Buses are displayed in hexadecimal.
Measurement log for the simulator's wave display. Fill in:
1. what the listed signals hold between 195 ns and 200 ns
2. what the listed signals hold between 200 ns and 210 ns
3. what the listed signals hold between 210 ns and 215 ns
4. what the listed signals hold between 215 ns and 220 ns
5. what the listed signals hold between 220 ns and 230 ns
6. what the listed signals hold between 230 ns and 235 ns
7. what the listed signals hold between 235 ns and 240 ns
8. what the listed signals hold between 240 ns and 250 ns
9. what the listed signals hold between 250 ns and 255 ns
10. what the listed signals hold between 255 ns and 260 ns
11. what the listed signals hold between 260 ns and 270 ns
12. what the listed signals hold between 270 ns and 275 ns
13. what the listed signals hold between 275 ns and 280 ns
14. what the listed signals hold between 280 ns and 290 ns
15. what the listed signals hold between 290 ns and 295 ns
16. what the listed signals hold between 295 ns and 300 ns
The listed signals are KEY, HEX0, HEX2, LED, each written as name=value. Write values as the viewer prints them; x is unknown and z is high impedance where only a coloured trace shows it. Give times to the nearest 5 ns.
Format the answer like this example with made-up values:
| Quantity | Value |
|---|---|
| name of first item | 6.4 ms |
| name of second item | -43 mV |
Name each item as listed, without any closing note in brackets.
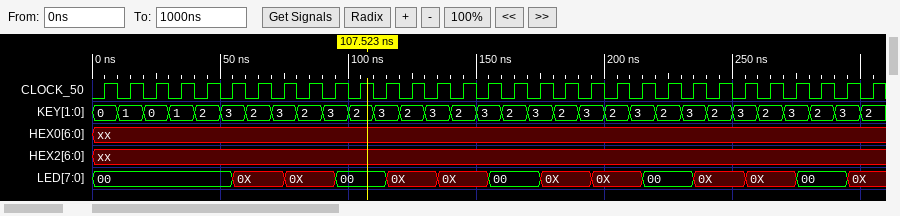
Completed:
| Quantity | Value |
|---|---|
| what the listed signals hold between 195 ns and 200 ns | KEY=3, HEX0=xx, HEX2=xx, LED=0X |
| what the listed signals hold between 200 ns and 210 ns | KEY=2, HEX0=xx, HEX2=xx, LED=0X |
| what the listed signals hold between 210 ns and 215 ns | KEY=3, HEX0=xx, HEX2=xx, LED=0X |
| what the listed signals hold between 215 ns and 220 ns | KEY=3, HEX0=xx, HEX2=xx, LED=00 |
| what the listed signals hold between 220 ns and 230 ns | KEY=2, HEX0=xx, HEX2=xx, LED=00 |
| what the listed signals hold between 230 ns and 235 ns | KEY=3, HEX0=xx, HEX2=xx, LED=00 |
| what the listed signals hold between 235 ns and 240 ns | KEY=3, HEX0=xx, HEX2=xx, LED=0X |
| what the listed signals hold between 240 ns and 250 ns | KEY=2, HEX0=xx, HEX2=xx, LED=0X |
| what the listed signals hold between 250 ns and 255 ns | KEY=3, HEX0=xx, HEX2=xx, LED=0X |
| what the listed signals hold between 255 ns and 260 ns | KEY=3, HEX0=xx, HEX2=xx, LED=0X |
| what the listed signals hold between 260 ns and 270 ns | KEY=2, HEX0=xx, HEX2=xx, LED=0X |
| what the listed signals hold between 270 ns and 275 ns | KEY=3, HEX0=xx, HEX2=xx, LED=0X |
| what the listed signals hold between 275 ns and 280 ns | KEY=3, HEX0=xx, HEX2=xx, LED=00 |
| what the listed signals hold between 280 ns and 290 ns | KEY=2, HEX0=xx, HEX2=xx, LED=00 |
| what the listed signals hold between 290 ns and 295 ns | KEY=3, HEX0=xx, HEX2=xx, LED=00 |
| what the listed signals hold between 295 ns and 300 ns | KEY=3, HEX0=xx, HEX2=xx, LED=0X |
